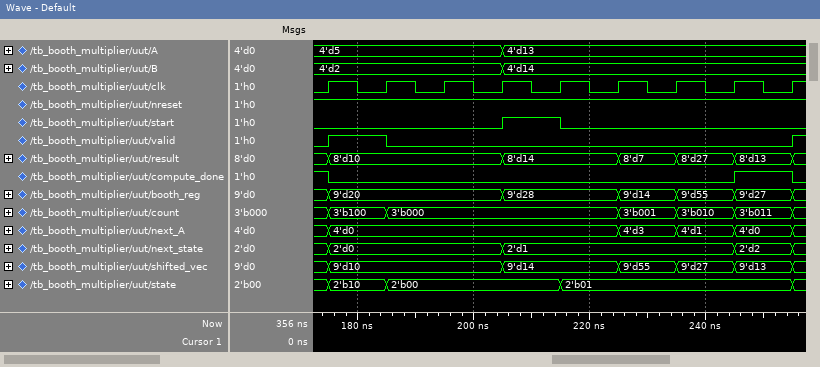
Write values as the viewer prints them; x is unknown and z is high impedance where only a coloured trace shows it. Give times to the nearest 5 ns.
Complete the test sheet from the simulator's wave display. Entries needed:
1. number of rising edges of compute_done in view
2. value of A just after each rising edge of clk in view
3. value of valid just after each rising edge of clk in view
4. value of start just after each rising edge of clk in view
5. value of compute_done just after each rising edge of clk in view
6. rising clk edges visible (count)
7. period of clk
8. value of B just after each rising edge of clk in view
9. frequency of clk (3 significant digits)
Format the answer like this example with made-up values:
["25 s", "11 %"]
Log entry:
["1", "4'd5, 4'd5, 4'd5, 4'd13, 4'd13, 4'd13, 4'd13, 4'd13, 4'd13", "1 0 0 0 0 0 0 0 1", "0 0 0 1 0 0 0 0 0", "0 0 0 0 0 0 0 1 0", "9", "10 ns", "4'd2, 4'd2, 4'd2, 4'd14, 4'd14, 4'd14, 4'd14, 4'd14, 4'd14", "100 MHz"]
